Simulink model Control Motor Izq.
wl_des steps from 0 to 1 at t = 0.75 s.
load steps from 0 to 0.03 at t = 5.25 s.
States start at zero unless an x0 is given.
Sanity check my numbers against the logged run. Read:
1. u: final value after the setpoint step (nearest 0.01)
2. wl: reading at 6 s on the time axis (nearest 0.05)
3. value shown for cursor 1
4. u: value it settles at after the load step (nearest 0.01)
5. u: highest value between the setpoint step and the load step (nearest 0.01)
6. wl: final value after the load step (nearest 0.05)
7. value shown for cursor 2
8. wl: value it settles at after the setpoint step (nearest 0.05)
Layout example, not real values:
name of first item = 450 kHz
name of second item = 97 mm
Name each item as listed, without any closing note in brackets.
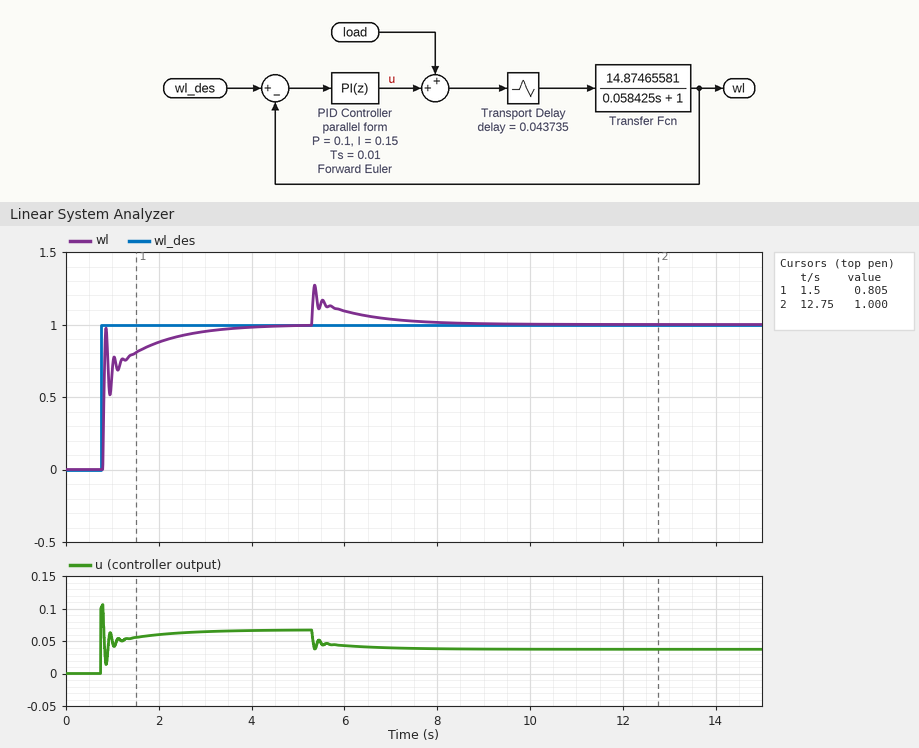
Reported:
u: final value after the setpoint step = 0.07
wl: reading at 6 s on the time axis = 1.10
value shown for cursor 1 = 0.805
u: value it settles at after the load step = 0.04
u: highest value between the setpoint step and the load step = 0.11
wl: final value after the load step = 1.00
value shown for cursor 2 = 1.000
wl: value it settles at after the setpoint step = 1.00
